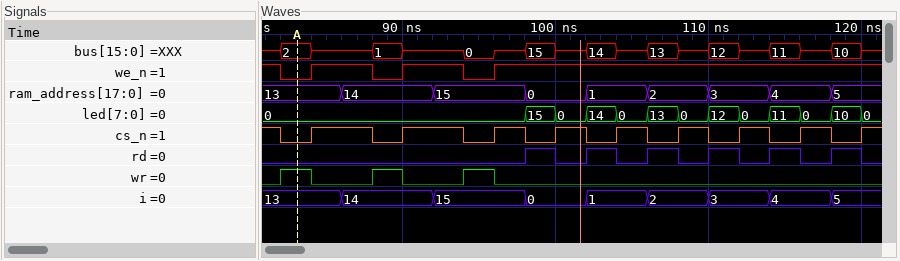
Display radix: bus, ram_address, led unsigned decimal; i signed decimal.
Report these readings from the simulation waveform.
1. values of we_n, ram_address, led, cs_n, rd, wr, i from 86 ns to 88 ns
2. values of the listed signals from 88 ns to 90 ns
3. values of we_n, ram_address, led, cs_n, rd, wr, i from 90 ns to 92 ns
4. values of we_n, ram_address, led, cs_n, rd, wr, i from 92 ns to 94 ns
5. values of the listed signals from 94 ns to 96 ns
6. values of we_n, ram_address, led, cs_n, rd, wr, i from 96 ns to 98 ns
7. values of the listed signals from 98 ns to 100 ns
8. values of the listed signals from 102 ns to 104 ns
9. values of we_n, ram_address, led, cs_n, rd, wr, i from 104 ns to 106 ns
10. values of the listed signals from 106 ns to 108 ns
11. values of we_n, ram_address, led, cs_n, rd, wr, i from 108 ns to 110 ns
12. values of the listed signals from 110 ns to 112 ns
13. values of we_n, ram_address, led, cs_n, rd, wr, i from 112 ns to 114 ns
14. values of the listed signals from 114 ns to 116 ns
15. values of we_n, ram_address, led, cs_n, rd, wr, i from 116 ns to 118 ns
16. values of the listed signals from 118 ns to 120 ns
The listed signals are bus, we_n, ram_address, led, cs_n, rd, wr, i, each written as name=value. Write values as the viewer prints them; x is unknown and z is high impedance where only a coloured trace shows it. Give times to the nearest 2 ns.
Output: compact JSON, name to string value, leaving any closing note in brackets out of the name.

{"values of we_n, ram_address, led, cs_n, rd, wr, i from 86 ns to 88 ns": "we_n=1, ram_address=14, led=0, cs_n=1, rd=0, wr=0, i=14", "values of the listed signals from 88 ns to 90 ns": "bus=1, we_n=0, ram_address=14, led=0, cs_n=0, rd=0, wr=1, i=14", "values of we_n, ram_address, led, cs_n, rd, wr, i from 90 ns to 92 ns": "we_n=1, ram_address=14, led=0, cs_n=1, rd=0, wr=0, i=14", "values of we_n, ram_address, led, cs_n, rd, wr, i from 92 ns to 94 ns": "we_n=1, ram_address=15, led=0, cs_n=1, rd=0, wr=0, i=15", "values of the listed signals from 94 ns to 96 ns": "bus=0, we_n=0, ram_address=15, led=0, cs_n=0, rd=0, wr=1, i=15", "values of we_n, ram_address, led, cs_n, rd, wr, i from 96 ns to 98 ns": "we_n=1, ram_address=15, led=0, cs_n=1, rd=0, wr=0, i=15", "values of the listed signals from 98 ns to 100 ns": "bus=15, we_n=1, ram_address=0, led=15, cs_n=0, rd=1, wr=0, i=0", "values of the listed signals from 102 ns to 104 ns": "bus=14, we_n=1, ram_address=1, led=14, cs_n=0, rd=1, wr=0, i=1", "values of we_n, ram_address, led, cs_n, rd, wr, i from 104 ns to 106 ns": "we_n=1, ram_address=1, led=0, cs_n=1, rd=0, wr=0, i=1", "values of the listed signals from 106 ns to 108 ns": "bus=13, we_n=1, ram_address=2, led=13, cs_n=0, rd=1, wr=0, i=2", "values of we_n, ram_address, led, cs_n, rd, wr, i from 108 ns to 110 ns": "we_n=1, ram_address=2, led=0, cs_n=1, rd=0, wr=0, i=2", "values of the listed signals from 110 ns to 112 ns": "bus=12, we_n=1, ram_address=3, led=12, cs_n=0, rd=1, wr=0, i=3", "values of we_n, ram_address, led, cs_n, rd, wr, i from 112 ns to 114 ns": "we_n=1, ram_address=3, led=0, cs_n=1, rd=0, wr=0, i=3", "values of the listed signals from 114 ns to 116 ns": "bus=11, we_n=1, ram_address=4, led=11, cs_n=0, rd=1, wr=0, i=4", "values of we_n, ram_address, led, cs_n, rd, wr, i from 116 ns to 118 ns": "we_n=1, ram_address=4, led=0, cs_n=1, rd=0, wr=0, i=4", "values of the listed signals from 118 ns to 120 ns": "bus=10, we_n=1, ram_address=5, led=10, cs_n=0, rd=1, wr=0, i=5"}
